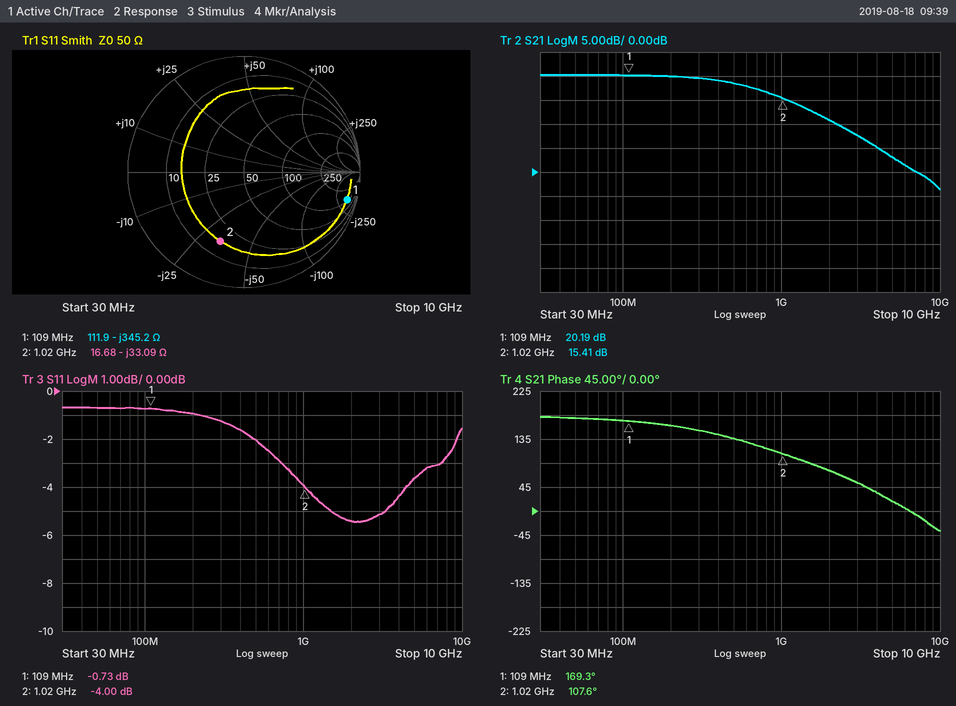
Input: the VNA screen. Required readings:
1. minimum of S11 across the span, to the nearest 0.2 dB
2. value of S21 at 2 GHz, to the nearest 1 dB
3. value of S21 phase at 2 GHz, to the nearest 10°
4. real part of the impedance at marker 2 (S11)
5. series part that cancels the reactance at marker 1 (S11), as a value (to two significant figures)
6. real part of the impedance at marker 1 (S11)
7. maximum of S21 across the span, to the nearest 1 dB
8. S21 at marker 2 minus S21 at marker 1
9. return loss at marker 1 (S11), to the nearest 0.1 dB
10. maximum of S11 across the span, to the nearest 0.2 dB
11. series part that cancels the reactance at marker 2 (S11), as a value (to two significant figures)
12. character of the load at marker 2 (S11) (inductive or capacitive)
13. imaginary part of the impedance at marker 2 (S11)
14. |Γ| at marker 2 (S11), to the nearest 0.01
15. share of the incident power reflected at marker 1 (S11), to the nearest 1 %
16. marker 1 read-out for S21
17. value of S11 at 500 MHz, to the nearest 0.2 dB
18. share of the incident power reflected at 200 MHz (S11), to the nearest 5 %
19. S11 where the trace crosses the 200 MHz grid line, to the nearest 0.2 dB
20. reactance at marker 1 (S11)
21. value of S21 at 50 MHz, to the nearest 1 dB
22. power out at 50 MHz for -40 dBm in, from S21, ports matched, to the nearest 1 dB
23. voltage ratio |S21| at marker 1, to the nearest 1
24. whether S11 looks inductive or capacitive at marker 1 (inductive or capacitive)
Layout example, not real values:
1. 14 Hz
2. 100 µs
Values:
1. -5.4 dB
2. 11 dB
3. 80°
4. 16.68 Ω
5. 500 nH
6. 111.9 Ω
7. 20 dB
8. -4.78 dB
9. 0.7 dB
10. -0.6 dB
11. 5.2 nH
12. capacitive
13. -33.09 Ω
14. 0.63
15. 85 %
16. 20.19 dB
17. -2.0 dB
18. 80 %
19. -1.0 dB
20. -345.2 Ω
21. 20 dB
22. -20 dBm
23. 10
24. capacitive
